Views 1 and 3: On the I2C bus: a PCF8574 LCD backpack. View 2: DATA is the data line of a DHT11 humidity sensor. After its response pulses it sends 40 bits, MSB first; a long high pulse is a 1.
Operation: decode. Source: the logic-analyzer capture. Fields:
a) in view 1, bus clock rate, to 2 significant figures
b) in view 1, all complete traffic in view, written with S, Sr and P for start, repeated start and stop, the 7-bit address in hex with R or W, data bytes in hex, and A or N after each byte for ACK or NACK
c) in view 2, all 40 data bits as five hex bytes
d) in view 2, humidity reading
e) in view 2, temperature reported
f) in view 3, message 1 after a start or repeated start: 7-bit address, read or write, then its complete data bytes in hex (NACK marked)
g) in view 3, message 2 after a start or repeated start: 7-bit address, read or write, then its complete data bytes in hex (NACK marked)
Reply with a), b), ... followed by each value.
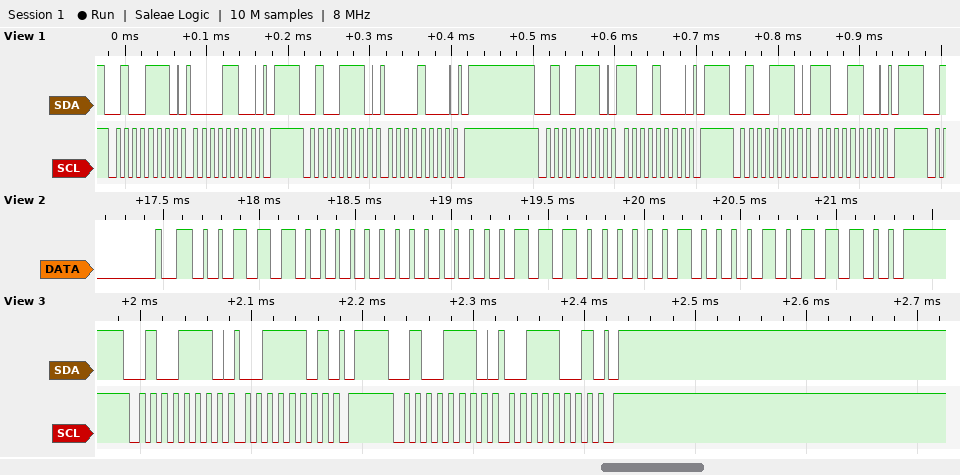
a) 100 kHz
b) S 27W A 0C A P S 27W A 08 A P S 27W A C8 A P S 27W A CC A P
c) 38 00 1C 08 5C
d) 56 %
e) 28.8 °C
f) 0x27 write: 3D
g) 0x27 write: 39
